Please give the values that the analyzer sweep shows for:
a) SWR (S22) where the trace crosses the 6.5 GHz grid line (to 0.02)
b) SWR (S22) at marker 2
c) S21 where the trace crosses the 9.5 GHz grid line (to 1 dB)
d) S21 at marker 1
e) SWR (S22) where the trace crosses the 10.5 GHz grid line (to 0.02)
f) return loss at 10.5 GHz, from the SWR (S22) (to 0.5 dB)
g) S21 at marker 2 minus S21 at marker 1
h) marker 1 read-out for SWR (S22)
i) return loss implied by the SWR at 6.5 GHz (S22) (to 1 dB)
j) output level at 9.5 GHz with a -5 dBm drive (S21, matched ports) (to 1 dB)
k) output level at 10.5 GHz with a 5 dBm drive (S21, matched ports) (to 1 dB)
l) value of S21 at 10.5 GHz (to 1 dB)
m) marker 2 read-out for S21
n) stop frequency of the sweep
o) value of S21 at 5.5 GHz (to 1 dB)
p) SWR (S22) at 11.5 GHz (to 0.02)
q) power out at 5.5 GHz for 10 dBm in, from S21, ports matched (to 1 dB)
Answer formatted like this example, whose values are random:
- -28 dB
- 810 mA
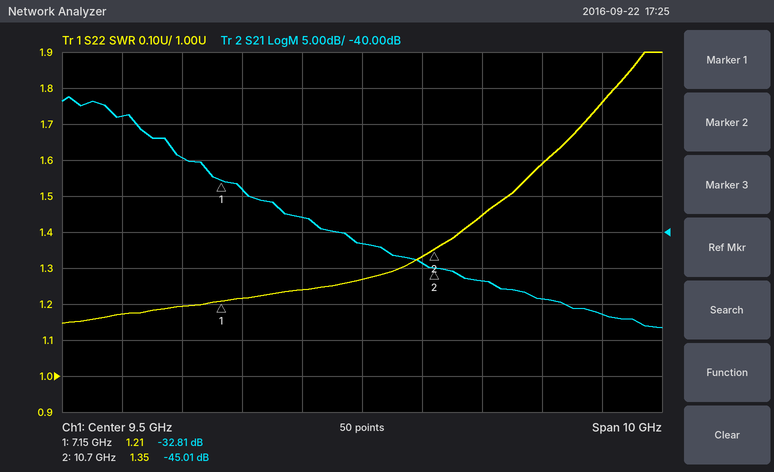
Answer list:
- 1.20
- 1.35
- -42 dB
- -32.81 dB
- 1.34
- 17.0 dB
- -12.20 dB
- 1.21
- 21 dB
- -47 dBm
- -39 dBm
- -44 dB
- -45.01 dB
- 14.5 GHz
- -24 dB
- 1.44
- -14 dBm
